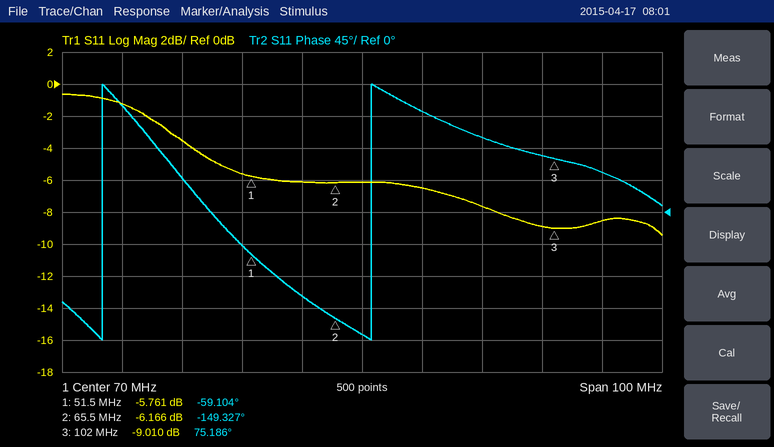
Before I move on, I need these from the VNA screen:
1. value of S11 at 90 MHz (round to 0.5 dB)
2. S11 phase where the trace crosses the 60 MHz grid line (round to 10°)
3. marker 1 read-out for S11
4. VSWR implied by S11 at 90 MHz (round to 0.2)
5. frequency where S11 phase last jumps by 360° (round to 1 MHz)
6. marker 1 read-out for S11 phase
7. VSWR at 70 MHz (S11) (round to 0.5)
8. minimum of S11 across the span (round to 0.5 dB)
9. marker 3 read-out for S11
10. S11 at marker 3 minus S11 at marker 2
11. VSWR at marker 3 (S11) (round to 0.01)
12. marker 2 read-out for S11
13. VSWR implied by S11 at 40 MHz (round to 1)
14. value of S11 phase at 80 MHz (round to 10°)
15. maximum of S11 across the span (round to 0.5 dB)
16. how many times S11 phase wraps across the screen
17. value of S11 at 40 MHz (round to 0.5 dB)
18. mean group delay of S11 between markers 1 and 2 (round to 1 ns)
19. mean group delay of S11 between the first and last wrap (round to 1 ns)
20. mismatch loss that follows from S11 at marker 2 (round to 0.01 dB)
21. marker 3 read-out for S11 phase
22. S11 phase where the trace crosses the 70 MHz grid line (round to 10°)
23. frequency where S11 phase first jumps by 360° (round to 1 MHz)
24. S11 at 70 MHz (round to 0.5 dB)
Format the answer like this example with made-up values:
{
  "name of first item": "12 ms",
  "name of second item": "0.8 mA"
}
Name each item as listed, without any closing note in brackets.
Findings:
{
  "value of S11 at 90 MHz": "-7.5 dB",
  "S11 phase where the trace crosses the 60 MHz grid line": "-120°",
  "marker 1 read-out for S11": "-5.761 dB",
  "VSWR implied by S11 at 90 MHz": "2.4",
  "frequency where S11 phase last jumps by 360°": "72 MHz",
  "marker 1 read-out for S11 phase": "-59.104°",
  "VSWR at 70 MHz (S11)": "3.0",
  "minimum of S11 across the span": "-9.5 dB",
  "marker 3 read-out for S11": "-9.010 dB",
  "S11 at marker 3 minus S11 at marker 2": "-2.844 dB",
  "VSWR at marker 3 (S11)": "2.10",
  "marker 2 read-out for S11": "-6.166 dB",
  "VSWR implied by S11 at 40 MHz": "5",
  "value of S11 phase at 80 MHz": "140°",
  "maximum of S11 across the span": "-0.5 dB",
  "how many times S11 phase wraps across the screen": "2",
  "value of S11 at 40 MHz": "-3.5 dB",
  "mean group delay of S11 between markers 1 and 2": "18 ns",
  "mean group delay of S11 between the first and last wrap": "22 ns",
  "mismatch loss that follows from S11 at marker 2": "1.20 dB",
  "marker 3 read-out for S11 phase": "75.186°",
  "S11 phase where the trace crosses the 70 MHz grid line": "-170°",
  "frequency where S11 phase first jumps by 360°": "27 MHz",
  "S11 at 70 MHz": "-6.0 dB"
}
